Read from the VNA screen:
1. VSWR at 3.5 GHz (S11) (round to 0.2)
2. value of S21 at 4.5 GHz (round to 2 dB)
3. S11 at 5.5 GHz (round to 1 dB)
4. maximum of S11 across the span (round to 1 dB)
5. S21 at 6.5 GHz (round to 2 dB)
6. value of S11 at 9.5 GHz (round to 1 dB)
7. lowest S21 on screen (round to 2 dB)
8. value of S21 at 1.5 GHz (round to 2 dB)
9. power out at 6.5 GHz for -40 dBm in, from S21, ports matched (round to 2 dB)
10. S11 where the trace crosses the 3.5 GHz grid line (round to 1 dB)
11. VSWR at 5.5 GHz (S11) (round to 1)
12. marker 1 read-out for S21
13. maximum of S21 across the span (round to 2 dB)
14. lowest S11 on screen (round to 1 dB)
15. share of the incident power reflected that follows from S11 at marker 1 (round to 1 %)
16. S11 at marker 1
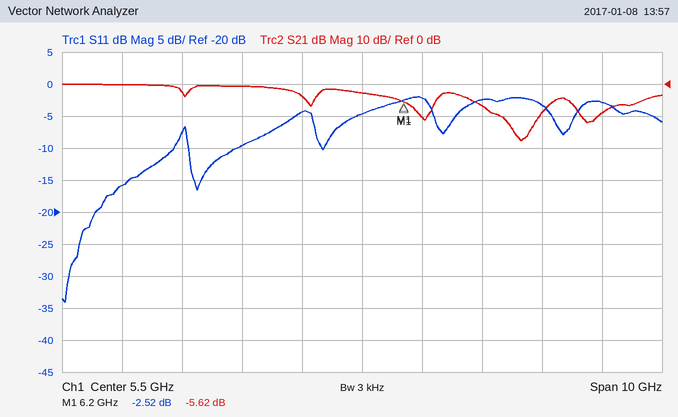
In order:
2.0
-4 dB
-5 dB
-2 dB
-10 dB
-3 dB
-18 dB
0 dB
-50 dBm
-10 dB
4
-5.62 dB
0 dB
-34 dB
56 %
-2.52 dB
